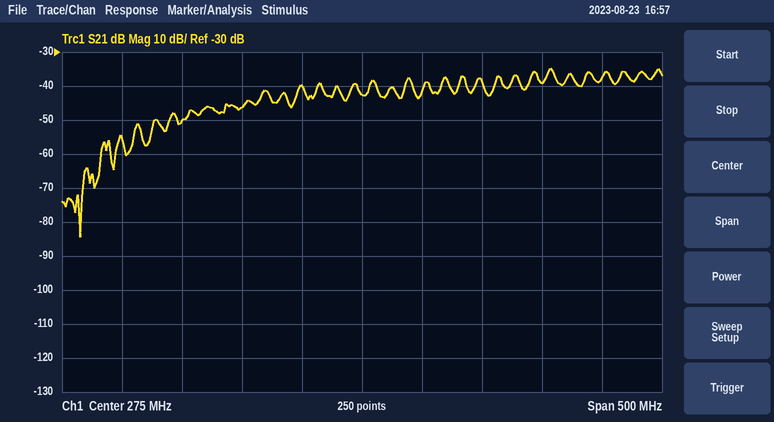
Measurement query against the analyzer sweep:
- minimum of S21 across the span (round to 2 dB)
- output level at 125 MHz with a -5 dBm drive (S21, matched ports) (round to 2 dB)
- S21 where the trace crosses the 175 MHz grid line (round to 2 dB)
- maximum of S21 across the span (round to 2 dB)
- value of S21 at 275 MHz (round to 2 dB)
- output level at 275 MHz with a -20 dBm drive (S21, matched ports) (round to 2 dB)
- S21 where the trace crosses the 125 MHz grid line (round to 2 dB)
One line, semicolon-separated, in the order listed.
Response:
-84 dB; -56 dBm; -46 dB; -34 dB; -42 dB; -62 dBm; -50 dB
